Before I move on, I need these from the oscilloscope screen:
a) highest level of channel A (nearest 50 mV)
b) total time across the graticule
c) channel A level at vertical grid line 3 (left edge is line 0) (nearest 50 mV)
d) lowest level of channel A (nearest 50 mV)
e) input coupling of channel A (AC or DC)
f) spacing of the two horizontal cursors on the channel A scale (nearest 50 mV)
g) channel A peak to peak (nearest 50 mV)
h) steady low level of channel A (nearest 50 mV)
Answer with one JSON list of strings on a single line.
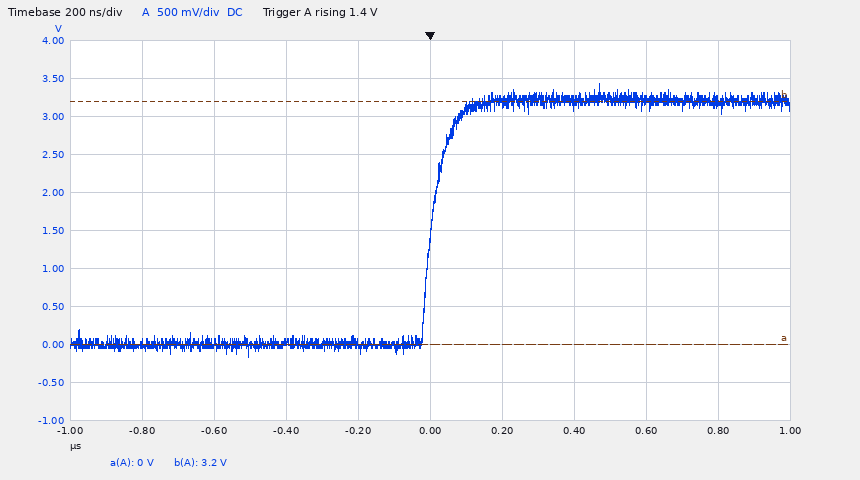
["3.45 V", "2 µs", "50 mV", "-150 mV", "DC", "3.20 V", "3.60 V", "0 mV"]
